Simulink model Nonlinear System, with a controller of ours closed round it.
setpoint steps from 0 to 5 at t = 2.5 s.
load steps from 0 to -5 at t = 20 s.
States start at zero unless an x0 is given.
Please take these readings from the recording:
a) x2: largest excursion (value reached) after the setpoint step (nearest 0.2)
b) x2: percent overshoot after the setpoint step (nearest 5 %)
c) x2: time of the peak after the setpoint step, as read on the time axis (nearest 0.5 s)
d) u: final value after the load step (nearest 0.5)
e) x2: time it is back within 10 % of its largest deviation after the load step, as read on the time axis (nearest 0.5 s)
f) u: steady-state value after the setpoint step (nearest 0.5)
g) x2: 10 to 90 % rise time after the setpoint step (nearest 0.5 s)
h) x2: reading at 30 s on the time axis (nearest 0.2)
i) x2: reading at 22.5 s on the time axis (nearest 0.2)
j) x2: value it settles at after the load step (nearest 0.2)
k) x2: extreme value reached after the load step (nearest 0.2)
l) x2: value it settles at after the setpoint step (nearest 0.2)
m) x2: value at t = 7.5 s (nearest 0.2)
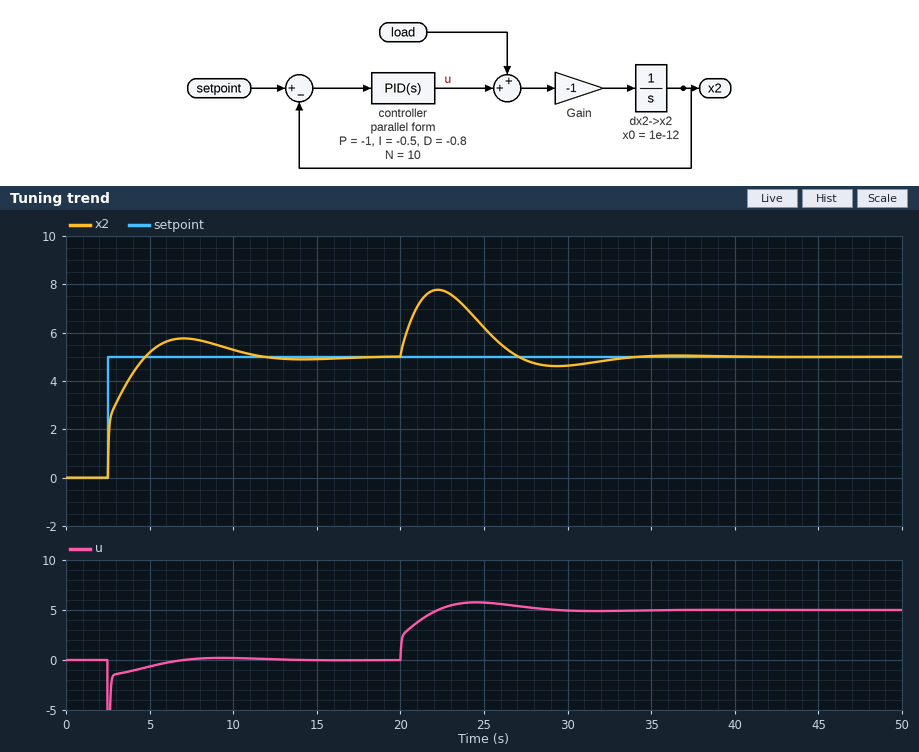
5.8
15 %
7.0 s
5.0
31.0 s
0.0
1.5 s
4.6
7.8
5.0
7.8
5.0
5.8
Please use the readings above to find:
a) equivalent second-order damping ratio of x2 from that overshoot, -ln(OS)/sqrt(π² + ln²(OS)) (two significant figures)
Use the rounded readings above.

0.52
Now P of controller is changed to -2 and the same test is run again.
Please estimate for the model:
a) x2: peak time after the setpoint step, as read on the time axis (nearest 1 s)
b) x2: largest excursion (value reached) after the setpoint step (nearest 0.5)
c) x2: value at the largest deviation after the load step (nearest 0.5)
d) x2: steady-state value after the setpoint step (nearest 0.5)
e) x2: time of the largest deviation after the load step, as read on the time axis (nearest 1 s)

6 s
5.5
7.0
5.0
22 s
